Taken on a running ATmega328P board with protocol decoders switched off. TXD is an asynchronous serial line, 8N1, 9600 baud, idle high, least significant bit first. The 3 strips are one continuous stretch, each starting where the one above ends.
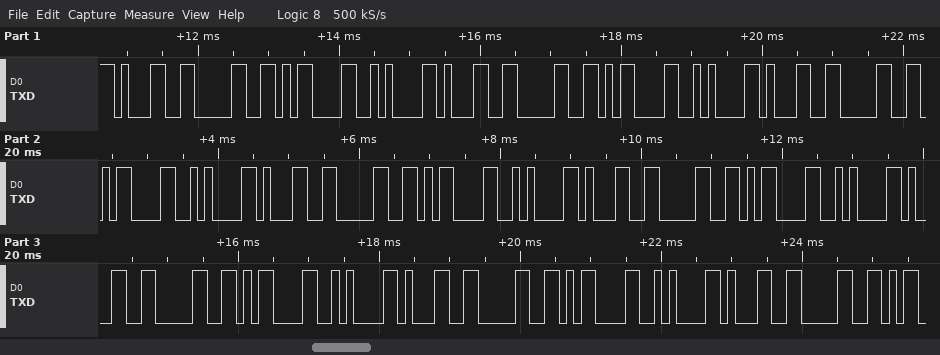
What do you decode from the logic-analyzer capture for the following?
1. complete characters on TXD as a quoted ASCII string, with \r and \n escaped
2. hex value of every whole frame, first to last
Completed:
"10\r\n10\r\n10\r\n10\r\n10\r\n10\r\n10\r\n10"
31 30 0D 0A 31 30 0D 0A 31 30 0D 0A 31 30 0D 0A 31 30 0D 0A 31 30 0D 0A 31 30 0D 0A 31 30
